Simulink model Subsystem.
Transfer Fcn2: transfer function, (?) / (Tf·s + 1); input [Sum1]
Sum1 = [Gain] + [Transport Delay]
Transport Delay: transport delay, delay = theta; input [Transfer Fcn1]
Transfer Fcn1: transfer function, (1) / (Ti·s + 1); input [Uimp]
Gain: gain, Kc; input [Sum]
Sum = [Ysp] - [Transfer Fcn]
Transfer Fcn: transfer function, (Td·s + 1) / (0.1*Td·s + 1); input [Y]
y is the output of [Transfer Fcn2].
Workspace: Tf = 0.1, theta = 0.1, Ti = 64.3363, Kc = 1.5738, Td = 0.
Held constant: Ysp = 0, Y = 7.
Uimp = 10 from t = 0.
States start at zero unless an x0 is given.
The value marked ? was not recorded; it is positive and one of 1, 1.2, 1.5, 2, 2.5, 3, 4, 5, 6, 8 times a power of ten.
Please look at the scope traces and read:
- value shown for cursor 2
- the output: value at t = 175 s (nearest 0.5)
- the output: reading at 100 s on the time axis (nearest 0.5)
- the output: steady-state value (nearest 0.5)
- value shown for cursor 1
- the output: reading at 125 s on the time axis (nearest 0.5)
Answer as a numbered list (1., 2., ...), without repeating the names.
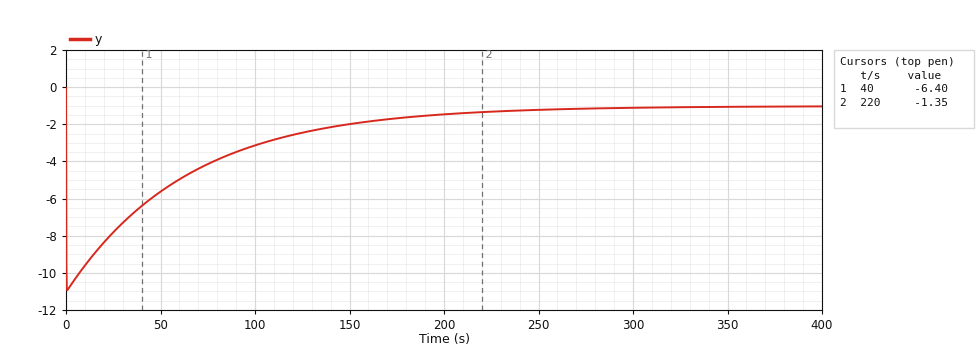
1. -1.35
2. -1.5
3. -3.0
4. -1.0
5. -6.40
6. -2.5
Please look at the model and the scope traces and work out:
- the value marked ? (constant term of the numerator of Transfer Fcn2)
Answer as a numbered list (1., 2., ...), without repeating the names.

1. 1
